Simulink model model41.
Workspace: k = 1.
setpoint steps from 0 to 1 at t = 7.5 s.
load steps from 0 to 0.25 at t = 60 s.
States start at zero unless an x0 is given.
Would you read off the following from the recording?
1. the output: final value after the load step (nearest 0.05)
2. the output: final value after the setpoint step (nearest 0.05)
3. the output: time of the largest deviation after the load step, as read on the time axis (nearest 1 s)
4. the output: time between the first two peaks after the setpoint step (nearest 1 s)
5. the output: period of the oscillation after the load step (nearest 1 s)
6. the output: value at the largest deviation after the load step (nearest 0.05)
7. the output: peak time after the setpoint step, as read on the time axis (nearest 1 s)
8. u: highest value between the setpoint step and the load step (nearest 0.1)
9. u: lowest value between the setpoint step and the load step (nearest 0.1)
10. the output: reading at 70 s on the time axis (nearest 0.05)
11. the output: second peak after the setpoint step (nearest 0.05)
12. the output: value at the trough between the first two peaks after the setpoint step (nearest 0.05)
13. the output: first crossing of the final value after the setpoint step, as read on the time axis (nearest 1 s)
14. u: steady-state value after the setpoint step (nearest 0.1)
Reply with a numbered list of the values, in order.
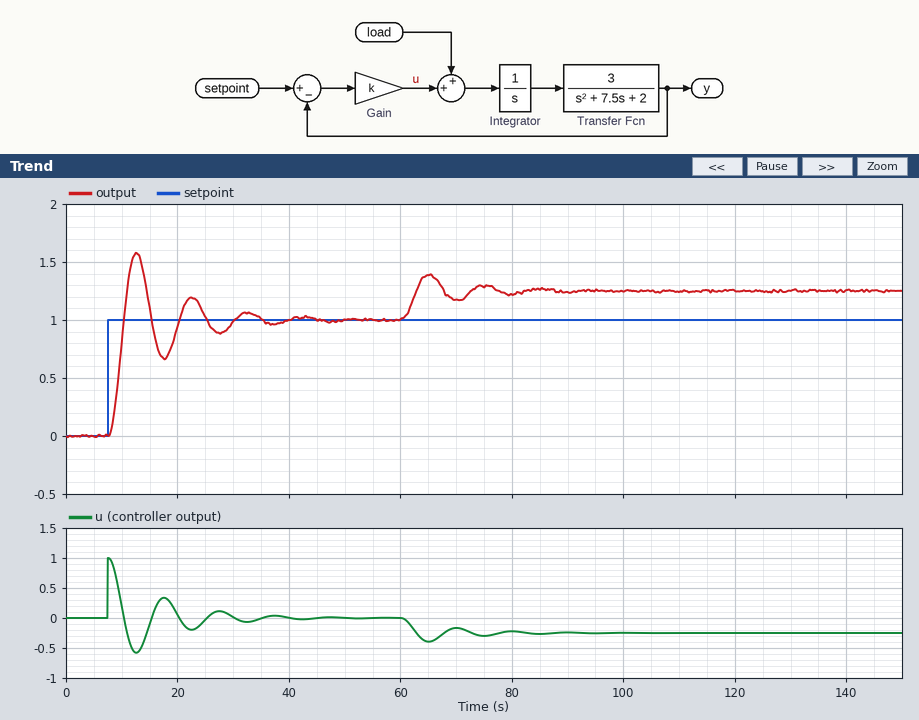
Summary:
1. 1.25
2. 1.00
3. 65 s
4. 10 s
5. 10 s
6. 1.40
7. 13 s
8. 1.0
9. -0.6
10. 1.15
11. 1.20
12. 0.65
13. 10 s
14. 0.0
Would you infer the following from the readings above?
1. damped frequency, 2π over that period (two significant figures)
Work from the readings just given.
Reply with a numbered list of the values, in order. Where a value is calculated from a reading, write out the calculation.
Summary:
1. 2π / 10 = 0.63 rad/s
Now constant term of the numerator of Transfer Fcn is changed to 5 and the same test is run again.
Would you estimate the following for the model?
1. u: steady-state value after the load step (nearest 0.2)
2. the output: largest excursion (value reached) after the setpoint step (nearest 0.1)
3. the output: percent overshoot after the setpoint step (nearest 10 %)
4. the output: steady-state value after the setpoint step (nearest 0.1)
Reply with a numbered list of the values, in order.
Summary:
1. -0.2
2. 1.7
3. 70 %
4. 1.0
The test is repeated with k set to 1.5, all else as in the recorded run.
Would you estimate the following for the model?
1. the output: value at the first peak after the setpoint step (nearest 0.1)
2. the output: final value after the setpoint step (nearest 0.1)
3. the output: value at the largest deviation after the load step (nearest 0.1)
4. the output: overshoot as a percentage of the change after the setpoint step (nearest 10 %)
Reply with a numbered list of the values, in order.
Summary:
1. 1.7
2. 1.0
3. 1.3
4. 70 %
